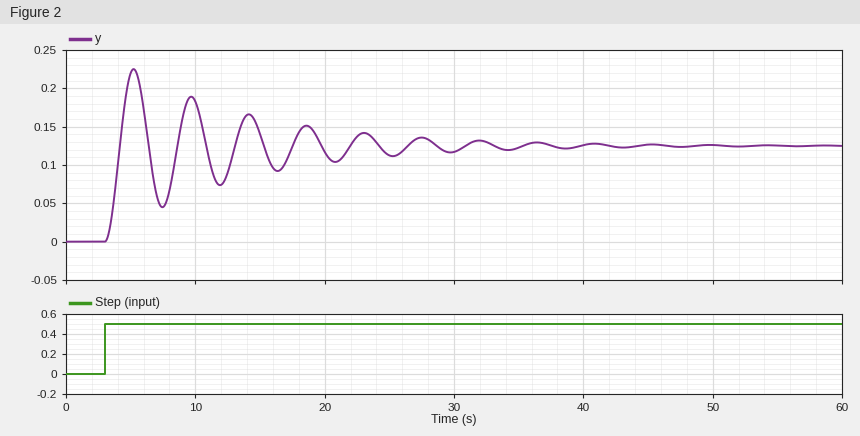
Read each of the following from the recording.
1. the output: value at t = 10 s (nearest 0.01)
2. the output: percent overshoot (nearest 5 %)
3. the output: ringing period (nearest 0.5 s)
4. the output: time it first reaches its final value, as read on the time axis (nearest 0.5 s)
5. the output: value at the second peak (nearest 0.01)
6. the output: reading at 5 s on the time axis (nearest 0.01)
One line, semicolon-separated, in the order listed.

0.18; 80 %; 4.5 s; 4.0 s; 0.19; 0.22
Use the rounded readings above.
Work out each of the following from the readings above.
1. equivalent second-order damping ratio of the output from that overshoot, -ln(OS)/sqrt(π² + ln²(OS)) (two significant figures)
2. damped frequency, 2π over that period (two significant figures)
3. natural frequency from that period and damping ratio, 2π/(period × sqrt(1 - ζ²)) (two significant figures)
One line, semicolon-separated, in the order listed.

0.071; 1.4 rad/s; 1.4 rad/s
